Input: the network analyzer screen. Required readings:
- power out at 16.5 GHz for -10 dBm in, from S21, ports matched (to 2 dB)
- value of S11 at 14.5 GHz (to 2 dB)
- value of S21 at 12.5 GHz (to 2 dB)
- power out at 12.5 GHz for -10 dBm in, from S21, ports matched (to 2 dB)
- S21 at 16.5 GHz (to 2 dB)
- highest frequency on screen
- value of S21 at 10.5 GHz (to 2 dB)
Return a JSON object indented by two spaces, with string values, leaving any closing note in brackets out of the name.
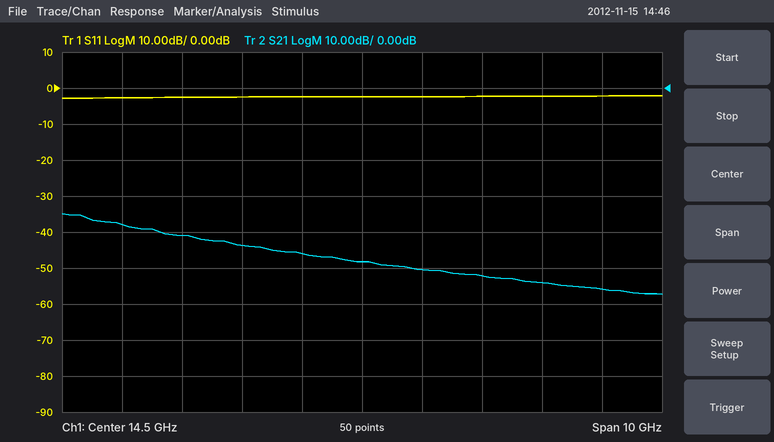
{
  "power out at 16.5 GHz for -10 dBm in, from S21, ports matched": "-62 dBm",
  "value of S11 at 14.5 GHz": "-2 dB",
  "value of S21 at 12.5 GHz": "-44 dB",
  "power out at 12.5 GHz for -10 dBm in, from S21, ports matched": "-54 dBm",
  "S21 at 16.5 GHz": "-52 dB",
  "highest frequency on screen": "19.5 GHz",
  "value of S21 at 10.5 GHz": "-38 dB"
}
